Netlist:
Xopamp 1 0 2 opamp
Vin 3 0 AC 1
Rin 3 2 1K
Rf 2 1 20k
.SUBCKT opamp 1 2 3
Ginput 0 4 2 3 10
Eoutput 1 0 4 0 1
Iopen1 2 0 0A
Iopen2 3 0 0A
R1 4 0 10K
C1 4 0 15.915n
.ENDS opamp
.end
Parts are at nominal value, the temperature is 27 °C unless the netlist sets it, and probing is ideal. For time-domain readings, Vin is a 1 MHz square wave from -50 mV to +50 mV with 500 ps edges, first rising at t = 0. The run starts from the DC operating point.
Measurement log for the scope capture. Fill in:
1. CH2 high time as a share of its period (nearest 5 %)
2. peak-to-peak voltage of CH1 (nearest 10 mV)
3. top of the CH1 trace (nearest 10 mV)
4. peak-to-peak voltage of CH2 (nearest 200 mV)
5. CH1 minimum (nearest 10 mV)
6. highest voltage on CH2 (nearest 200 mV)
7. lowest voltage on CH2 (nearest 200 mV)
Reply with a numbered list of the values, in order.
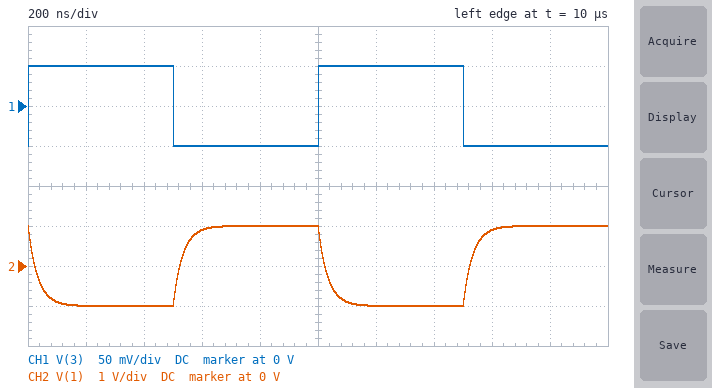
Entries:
1. 50 %
2. 100 mV
3. 50 mV
4. 2.0 V
5. -50 mV
6. 1.0 V
7. -1.0 V
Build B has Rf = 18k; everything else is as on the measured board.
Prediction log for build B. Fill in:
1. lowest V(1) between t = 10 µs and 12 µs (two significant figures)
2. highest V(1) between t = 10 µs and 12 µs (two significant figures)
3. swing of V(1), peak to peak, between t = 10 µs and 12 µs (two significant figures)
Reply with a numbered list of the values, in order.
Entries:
1. -900 mV
2. 900 mV
3. 1.8 V
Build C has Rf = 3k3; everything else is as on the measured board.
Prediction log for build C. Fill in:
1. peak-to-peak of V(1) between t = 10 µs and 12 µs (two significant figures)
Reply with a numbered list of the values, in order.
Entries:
1. 330 mV
